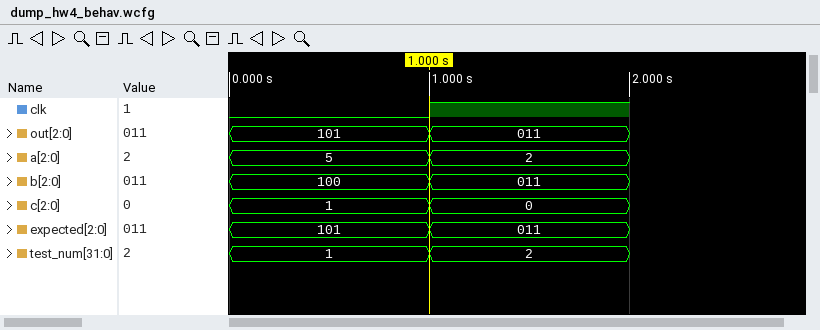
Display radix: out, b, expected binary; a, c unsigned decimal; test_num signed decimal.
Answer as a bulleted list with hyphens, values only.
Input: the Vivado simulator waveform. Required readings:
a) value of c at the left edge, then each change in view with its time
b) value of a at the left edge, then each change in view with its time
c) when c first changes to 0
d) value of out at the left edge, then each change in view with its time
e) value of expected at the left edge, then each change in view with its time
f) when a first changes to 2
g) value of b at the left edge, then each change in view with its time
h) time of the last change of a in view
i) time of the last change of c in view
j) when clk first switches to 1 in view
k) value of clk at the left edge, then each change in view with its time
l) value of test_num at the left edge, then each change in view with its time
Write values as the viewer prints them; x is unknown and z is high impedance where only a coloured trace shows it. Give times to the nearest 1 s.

- 1, 0 at 1 s
- 5, 2 at 1 s
- 1 s
- 101, 011 at 1 s
- 101, 011 at 1 s
- 1 s
- 100, 011 at 1 s
- 1 s
- 1 s
- 1 s
- 0, 1 at 1 s
- 1, 2 at 1 s
